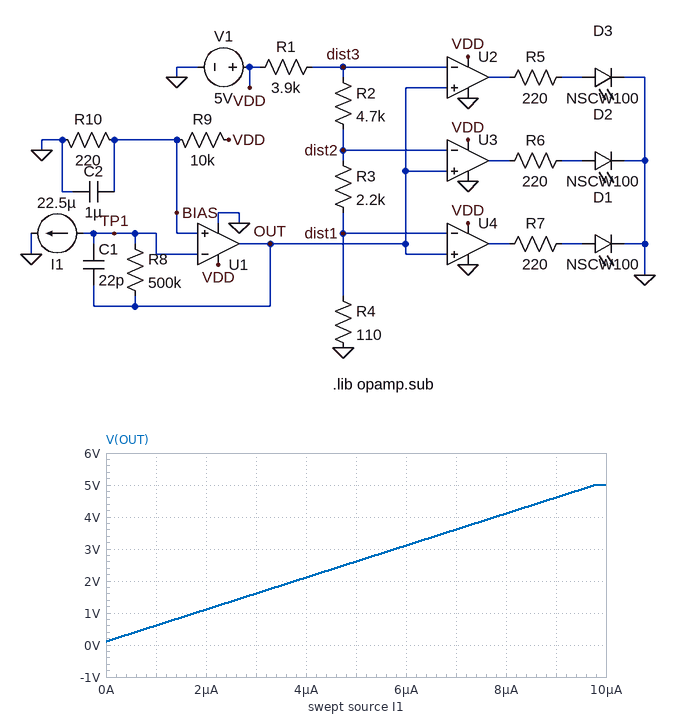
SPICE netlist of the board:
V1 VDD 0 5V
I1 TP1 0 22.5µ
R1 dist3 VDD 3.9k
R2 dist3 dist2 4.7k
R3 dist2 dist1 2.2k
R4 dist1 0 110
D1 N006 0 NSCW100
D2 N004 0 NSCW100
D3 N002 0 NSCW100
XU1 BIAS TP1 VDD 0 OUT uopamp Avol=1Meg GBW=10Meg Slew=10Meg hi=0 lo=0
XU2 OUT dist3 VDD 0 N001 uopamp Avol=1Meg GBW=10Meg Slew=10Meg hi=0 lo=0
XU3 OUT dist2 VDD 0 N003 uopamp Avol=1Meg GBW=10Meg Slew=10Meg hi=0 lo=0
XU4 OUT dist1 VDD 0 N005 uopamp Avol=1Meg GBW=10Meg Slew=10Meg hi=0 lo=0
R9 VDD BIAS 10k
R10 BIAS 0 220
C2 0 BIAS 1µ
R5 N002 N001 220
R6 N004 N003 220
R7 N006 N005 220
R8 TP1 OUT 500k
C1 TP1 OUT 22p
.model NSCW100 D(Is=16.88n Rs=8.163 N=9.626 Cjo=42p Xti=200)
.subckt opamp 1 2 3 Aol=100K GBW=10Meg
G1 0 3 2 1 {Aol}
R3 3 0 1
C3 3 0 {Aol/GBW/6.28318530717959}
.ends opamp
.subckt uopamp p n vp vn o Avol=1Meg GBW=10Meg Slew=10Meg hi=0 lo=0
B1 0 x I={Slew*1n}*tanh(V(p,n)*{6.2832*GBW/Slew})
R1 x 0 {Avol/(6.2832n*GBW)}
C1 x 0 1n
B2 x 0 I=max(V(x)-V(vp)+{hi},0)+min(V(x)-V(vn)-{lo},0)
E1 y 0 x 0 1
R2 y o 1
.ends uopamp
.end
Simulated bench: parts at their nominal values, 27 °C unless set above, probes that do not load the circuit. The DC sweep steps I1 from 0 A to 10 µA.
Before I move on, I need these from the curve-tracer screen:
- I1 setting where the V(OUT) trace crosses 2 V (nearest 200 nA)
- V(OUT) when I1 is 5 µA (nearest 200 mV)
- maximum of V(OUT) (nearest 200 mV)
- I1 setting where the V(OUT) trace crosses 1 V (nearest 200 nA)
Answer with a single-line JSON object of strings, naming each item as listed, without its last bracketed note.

{"I1 setting where the V(OUT) trace crosses 2 V": "3.8 µA", "V(OUT) when I1 is 5 µA": "2.6 V", "maximum of V(OUT)": "5.0 V", "I1 setting where the V(OUT) trace crosses 1 V": "1.8 µA"}
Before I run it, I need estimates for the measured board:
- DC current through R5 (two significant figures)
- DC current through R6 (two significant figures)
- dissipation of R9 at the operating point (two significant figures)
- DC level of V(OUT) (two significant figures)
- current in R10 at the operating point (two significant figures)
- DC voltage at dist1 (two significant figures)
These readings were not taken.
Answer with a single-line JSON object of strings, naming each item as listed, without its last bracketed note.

{"DC current through R5": "7.7 mA", "DC current through R6": "7.7 mA", "dissipation of R9 at the operating point": "2.4 mW", "DC level of V(OUT)": "5.0 V", "current in R10 at the operating point": "490 µA", "DC voltage at dist1": "50 mV"}
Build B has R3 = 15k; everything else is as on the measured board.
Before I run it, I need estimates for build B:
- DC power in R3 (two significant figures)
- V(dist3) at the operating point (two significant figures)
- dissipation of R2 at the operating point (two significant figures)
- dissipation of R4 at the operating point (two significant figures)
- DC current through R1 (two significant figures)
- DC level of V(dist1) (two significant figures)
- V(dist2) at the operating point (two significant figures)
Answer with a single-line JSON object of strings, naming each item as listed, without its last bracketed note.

{"DC power in R3": "670 µW", "V(dist3) at the operating point": "4.2 V", "dissipation of R2 at the operating point": "210 µW", "dissipation of R4 at the operating point": "4.9 µW", "DC current through R1": "210 µA", "DC level of V(dist1)": "23 mV", "V(dist2) at the operating point": "3.2 V"}
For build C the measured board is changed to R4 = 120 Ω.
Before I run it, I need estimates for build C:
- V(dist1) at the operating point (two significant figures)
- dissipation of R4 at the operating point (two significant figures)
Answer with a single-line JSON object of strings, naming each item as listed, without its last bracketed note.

{"V(dist1) at the operating point": "55 mV", "dissipation of R4 at the operating point": "25 µW"}
